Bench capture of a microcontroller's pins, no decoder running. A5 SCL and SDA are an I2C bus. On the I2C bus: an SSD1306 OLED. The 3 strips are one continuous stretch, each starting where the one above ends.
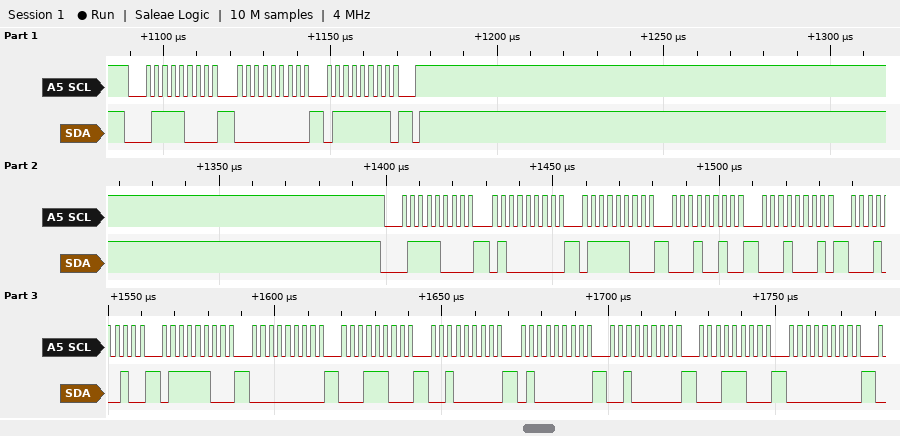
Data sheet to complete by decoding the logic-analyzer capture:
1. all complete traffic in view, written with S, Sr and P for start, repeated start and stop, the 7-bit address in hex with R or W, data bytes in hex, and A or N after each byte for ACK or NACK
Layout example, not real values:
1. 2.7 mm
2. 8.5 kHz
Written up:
1. S 3CW A 00 A 7F A P S 3CW A 40 A 7C A 12 A 11 A 12 A 7C A 00 A 1C A 20 A 40 A 20 A 1C A 00 A
